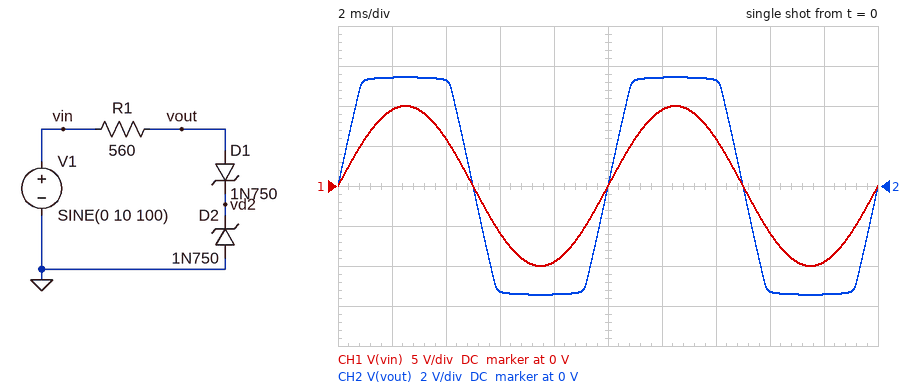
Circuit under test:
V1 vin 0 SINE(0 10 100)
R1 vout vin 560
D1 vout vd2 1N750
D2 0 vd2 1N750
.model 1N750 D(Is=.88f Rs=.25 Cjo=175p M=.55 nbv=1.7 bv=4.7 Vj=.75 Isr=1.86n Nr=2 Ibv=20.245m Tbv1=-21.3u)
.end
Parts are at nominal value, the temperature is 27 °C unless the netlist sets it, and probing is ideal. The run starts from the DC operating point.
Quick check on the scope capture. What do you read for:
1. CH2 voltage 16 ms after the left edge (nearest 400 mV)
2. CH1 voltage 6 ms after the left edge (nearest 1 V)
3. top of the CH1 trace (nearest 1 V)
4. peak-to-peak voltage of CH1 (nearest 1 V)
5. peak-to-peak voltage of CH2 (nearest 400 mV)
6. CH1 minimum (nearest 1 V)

-5.2 V
-6 V
10 V
20 V
10.8 V
-10 V
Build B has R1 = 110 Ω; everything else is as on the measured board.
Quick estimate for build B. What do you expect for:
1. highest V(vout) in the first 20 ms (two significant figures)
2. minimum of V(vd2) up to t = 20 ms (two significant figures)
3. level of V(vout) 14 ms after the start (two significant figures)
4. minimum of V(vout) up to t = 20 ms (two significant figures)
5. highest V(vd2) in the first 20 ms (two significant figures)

5.6 V
-820 mV
5.4 V
-5.6 V
4.7 V
